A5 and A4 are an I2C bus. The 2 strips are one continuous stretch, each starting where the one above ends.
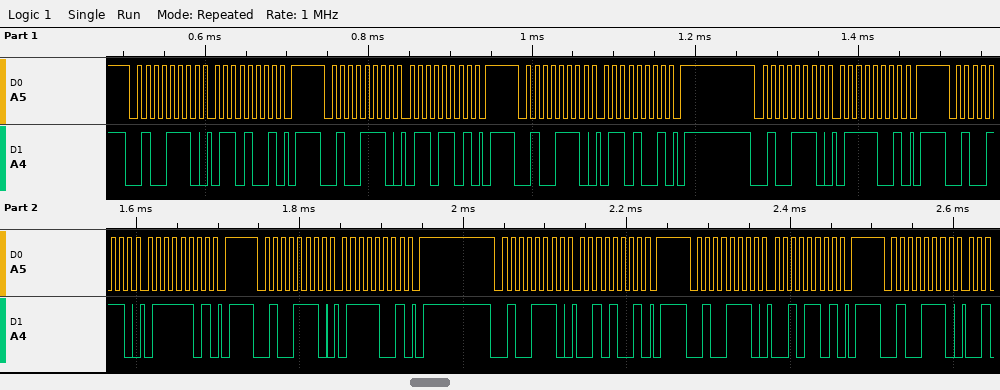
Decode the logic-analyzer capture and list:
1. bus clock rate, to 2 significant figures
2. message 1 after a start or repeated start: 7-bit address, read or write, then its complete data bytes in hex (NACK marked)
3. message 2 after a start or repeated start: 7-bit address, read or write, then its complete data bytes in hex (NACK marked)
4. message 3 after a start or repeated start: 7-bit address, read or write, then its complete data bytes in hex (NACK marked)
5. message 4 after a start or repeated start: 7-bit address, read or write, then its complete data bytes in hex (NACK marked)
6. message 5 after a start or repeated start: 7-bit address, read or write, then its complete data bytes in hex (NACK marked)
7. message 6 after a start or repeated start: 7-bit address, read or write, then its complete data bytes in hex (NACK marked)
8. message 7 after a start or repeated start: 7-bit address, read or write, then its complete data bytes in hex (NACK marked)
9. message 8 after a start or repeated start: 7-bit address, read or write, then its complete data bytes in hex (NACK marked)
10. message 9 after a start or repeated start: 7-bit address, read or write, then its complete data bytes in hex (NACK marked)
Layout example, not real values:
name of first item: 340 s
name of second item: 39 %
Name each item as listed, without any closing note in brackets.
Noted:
bus clock rate, to 2 significant figures: 100 kHz
message 1 after a start or repeated start: 7-bit address, read or write, then its complete data bytes in hex: 0x27 write: 69
message 2 after a start or repeated start: 7-bit address, read or write, then its complete data bytes in hex: 0x27 write: 6D
message 3 after a start or repeated start: 7-bit address, read or write, then its complete data bytes in hex: 0x27 write: 69
message 4 after a start or repeated start: 7-bit address, read or write, then its complete data bytes in hex: 0x27 write: 79
message 5 after a start or repeated start: 7-bit address, read or write, then its complete data bytes in hex: 0x27 write: 7D
message 6 after a start or repeated start: 7-bit address, read or write, then its complete data bytes in hex: 0x27 write: 79
message 7 after a start or repeated start: 7-bit address, read or write, then its complete data bytes in hex: 0x27 write: 29
message 8 after a start or repeated start: 7-bit address, read or write, then its complete data bytes in hex: 0x27 write: 2D
message 9 after a start or repeated start: 7-bit address, read or write, then its complete data bytes in hex: 0x27 write
